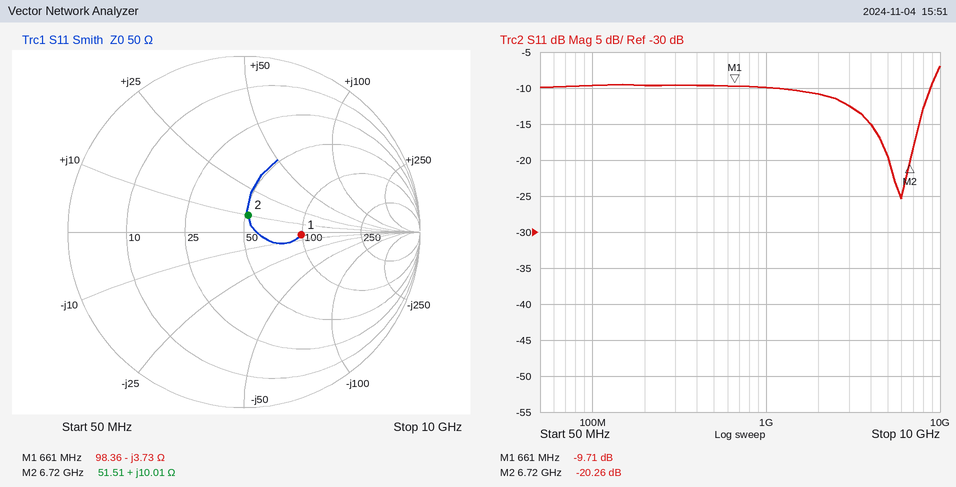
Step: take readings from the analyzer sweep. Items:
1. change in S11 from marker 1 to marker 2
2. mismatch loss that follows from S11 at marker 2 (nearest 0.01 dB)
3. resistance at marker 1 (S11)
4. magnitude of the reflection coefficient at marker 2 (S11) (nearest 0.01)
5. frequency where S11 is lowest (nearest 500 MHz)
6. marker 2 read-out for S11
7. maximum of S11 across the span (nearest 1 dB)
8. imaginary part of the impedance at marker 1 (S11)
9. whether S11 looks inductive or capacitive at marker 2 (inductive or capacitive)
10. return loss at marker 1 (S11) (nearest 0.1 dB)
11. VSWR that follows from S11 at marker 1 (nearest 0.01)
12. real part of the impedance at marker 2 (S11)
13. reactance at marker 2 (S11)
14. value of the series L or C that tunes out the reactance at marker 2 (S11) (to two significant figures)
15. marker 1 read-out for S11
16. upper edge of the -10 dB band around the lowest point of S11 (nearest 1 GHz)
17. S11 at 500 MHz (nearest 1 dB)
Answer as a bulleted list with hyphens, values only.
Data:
- -10.55 dB
- 0.04 dB
- 98.36 Ω
- 0.10
- 6.0 GHz
- -20.26 dB
- -7 dB
- -3.73 Ω
- inductive
- 9.7 dB
- 1.97
- 51.51 Ω
- +10.01 Ω
- 2.4 pF
- -9.71 dB
- 9 GHz
- -10 dB
